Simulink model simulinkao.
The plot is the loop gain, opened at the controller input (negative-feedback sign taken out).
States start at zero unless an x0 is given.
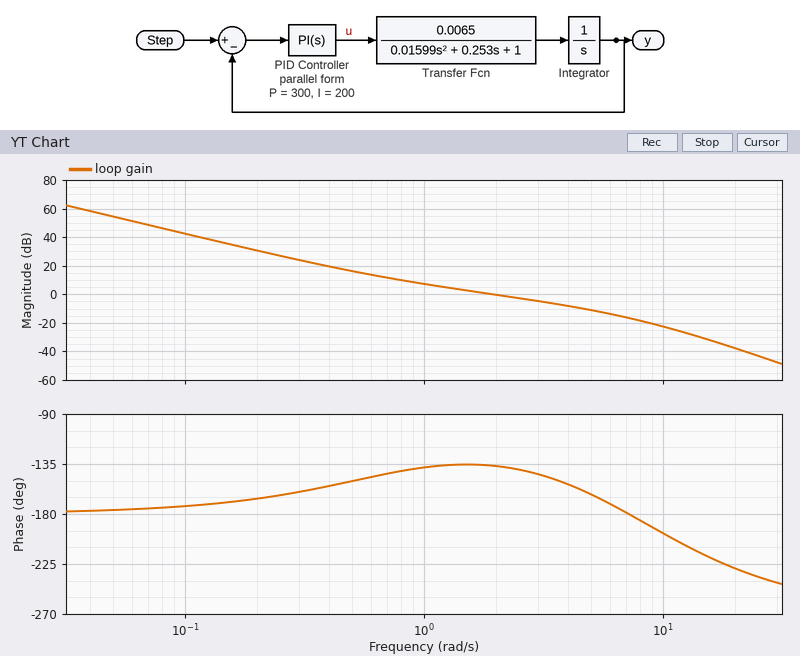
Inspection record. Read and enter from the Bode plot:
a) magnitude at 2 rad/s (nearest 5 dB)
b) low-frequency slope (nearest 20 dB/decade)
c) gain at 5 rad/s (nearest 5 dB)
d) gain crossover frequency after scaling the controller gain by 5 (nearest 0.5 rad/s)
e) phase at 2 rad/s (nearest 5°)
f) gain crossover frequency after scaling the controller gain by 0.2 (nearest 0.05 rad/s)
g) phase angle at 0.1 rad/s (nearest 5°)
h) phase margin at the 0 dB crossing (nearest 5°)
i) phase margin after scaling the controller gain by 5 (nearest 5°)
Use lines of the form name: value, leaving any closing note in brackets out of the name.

magnitude at 2 rad/s: 0 dB
low-frequency slope: -40 dB/decade
gain at 5 rad/s: -10 dB
gain crossover frequency after scaling the controller gain by 5: 6.0 rad/s
phase at 2 rad/s: -135°
gain crossover frequency after scaling the controller gain by 0.2: 0.60 rad/s
phase angle at 0.1 rad/s: -175°
phase margin at the 0 dB crossing: 45°
phase margin after scaling the controller gain by 5: 10°
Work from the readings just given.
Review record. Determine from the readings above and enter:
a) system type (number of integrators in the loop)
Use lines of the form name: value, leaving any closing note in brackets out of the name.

system type: 2
